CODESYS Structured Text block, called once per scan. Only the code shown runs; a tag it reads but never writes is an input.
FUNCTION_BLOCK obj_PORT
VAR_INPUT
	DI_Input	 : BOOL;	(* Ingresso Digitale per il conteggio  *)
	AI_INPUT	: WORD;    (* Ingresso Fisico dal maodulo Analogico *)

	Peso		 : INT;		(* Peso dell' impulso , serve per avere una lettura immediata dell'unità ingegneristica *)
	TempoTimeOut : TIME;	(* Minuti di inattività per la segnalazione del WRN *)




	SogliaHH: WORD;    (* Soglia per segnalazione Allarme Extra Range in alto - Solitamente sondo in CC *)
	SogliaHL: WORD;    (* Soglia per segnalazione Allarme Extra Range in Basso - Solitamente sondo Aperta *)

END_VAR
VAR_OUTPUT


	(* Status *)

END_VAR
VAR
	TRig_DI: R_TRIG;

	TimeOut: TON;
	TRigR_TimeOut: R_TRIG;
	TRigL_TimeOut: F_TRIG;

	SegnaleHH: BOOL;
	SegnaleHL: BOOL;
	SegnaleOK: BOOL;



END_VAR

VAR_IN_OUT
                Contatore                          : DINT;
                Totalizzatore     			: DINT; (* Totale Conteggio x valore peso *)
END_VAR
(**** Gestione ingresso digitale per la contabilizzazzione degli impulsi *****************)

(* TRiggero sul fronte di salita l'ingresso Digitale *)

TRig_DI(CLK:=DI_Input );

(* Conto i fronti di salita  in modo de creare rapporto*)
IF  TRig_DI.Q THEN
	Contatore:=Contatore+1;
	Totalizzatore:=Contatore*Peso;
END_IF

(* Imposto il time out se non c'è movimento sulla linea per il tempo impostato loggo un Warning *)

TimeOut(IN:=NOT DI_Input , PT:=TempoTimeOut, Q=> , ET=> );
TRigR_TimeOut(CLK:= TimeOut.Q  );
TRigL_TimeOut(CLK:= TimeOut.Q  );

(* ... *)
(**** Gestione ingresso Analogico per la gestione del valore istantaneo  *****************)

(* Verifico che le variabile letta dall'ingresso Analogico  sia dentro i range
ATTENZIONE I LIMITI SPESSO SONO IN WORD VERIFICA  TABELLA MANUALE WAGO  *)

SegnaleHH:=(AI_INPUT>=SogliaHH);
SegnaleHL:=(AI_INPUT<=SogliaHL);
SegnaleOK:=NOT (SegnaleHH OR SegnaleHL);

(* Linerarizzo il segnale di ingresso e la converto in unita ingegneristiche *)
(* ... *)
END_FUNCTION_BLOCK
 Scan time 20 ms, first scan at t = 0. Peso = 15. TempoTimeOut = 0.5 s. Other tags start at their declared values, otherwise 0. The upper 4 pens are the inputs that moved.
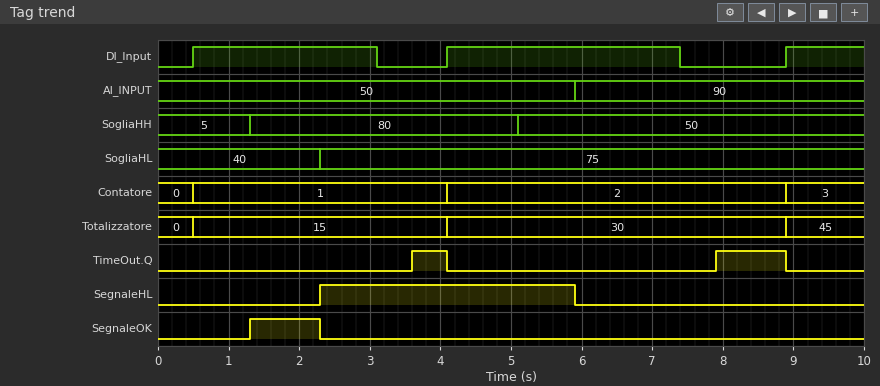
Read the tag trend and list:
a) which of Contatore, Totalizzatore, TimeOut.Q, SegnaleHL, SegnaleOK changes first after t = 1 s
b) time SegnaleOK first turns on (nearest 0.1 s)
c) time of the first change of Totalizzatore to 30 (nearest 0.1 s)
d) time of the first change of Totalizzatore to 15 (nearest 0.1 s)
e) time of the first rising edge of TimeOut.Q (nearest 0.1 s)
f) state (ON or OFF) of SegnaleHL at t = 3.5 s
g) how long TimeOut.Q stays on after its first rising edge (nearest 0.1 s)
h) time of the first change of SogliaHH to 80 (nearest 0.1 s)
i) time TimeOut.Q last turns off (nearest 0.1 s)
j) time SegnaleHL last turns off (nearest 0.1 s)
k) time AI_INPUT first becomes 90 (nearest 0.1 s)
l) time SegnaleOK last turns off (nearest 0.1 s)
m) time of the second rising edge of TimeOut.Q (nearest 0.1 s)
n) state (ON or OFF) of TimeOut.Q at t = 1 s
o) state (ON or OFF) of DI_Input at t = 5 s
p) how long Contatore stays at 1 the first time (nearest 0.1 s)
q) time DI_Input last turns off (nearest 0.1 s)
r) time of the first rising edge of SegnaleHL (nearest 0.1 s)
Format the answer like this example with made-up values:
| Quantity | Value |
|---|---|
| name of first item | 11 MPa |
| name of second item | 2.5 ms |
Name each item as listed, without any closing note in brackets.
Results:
| Quantity | Value |
|---|---|
| which of Contatore, Totalizzatore, TimeOut.Q, SegnaleHL, SegnaleOK changes first after t = 1 s | SegnaleOK |
| time SegnaleOK first turns on | 1.3 s |
| time of the first change of Totalizzatore to 30 | 4.1 s |
| time of the first change of Totalizzatore to 15 | 0.5 s |
| time of the first rising edge of TimeOut.Q | 3.6 s |
| state (ON or OFF) of SegnaleHL at t = 3.5 s | ON |
| how long TimeOut.Q stays on after its first rising edge | 0.5 s |
| time of the first change of SogliaHH to 80 | 1.3 s |
| time TimeOut.Q last turns off | 8.9 s |
| time SegnaleHL last turns off | 5.9 s |
| time AI_INPUT first becomes 90 | 5.9 s |
| time SegnaleOK last turns off | 2.3 s |
| time of the second rising edge of TimeOut.Q | 7.9 s |
| state (ON or OFF) of TimeOut.Q at t = 1 s | OFF |
| state (ON or OFF) of DI_Input at t = 5 s | ON |
| how long Contatore stays at 1 the first time | 3.6 s |
| time DI_Input last turns off | 7.4 s |
| time of the first rising edge of SegnaleHL | 2.3 s |
